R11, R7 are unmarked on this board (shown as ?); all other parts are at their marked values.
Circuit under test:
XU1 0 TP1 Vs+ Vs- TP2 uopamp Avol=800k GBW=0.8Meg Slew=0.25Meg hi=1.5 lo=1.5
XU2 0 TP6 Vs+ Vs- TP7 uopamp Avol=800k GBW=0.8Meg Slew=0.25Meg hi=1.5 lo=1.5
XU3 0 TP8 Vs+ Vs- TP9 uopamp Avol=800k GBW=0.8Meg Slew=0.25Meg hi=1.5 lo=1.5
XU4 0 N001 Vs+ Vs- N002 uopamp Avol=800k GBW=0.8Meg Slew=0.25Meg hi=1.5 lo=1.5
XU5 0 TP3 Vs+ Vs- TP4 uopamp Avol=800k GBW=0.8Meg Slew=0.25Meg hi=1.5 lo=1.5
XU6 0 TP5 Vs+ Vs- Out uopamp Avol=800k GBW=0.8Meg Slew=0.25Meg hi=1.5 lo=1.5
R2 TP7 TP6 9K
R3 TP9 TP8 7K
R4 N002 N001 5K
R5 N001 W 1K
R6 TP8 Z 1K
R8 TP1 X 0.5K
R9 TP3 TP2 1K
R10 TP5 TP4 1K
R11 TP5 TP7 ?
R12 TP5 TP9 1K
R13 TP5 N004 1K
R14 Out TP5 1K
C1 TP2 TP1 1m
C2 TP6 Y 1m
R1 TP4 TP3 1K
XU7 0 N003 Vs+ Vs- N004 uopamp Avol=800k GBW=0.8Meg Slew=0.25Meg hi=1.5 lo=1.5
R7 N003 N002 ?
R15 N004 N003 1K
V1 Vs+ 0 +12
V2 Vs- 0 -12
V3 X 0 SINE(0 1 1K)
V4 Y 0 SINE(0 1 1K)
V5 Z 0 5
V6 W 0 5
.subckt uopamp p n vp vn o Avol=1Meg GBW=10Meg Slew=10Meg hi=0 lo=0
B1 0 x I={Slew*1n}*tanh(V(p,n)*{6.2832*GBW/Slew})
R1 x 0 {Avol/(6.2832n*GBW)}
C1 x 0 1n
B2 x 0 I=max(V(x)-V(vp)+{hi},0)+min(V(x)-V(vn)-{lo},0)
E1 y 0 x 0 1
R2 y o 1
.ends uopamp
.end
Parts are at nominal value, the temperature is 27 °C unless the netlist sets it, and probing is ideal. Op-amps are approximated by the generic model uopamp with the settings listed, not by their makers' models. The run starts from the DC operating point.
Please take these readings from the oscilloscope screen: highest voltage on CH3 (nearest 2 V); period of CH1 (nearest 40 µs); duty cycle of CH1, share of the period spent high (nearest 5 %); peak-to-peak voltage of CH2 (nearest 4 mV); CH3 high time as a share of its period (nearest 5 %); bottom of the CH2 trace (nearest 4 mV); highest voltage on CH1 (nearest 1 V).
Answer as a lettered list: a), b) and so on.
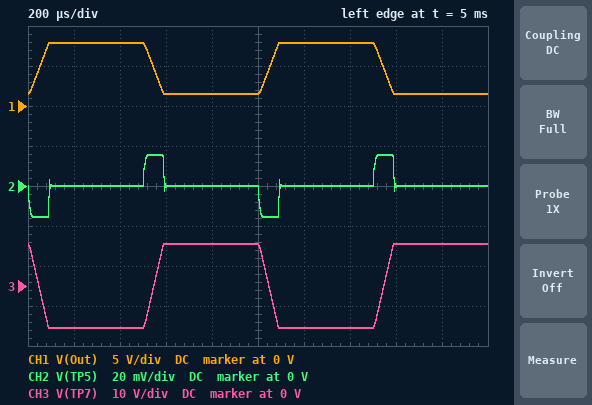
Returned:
a) 10 V
b) 1.00 ms
c) 50 %
d) 32 mV
e) 50 %
f) -16 mV
g) 8 V
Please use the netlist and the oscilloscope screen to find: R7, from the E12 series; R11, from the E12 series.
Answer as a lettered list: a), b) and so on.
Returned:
a) 1.8 kΩ
b) 3.3 kΩ
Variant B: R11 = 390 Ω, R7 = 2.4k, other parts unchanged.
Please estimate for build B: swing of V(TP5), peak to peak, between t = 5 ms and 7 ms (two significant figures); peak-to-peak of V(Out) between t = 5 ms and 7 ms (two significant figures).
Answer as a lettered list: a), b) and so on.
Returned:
a) 7.0 V
b) 21 V
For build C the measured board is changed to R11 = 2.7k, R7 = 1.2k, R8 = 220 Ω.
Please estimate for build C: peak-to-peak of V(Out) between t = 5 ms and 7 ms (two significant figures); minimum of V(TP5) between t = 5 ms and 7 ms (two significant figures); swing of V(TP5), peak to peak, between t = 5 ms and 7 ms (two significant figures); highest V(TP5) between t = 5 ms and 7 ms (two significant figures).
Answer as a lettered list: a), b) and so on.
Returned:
a) 7.8 V
b) -19 mV
c) 39 mV
d) 19 mV
